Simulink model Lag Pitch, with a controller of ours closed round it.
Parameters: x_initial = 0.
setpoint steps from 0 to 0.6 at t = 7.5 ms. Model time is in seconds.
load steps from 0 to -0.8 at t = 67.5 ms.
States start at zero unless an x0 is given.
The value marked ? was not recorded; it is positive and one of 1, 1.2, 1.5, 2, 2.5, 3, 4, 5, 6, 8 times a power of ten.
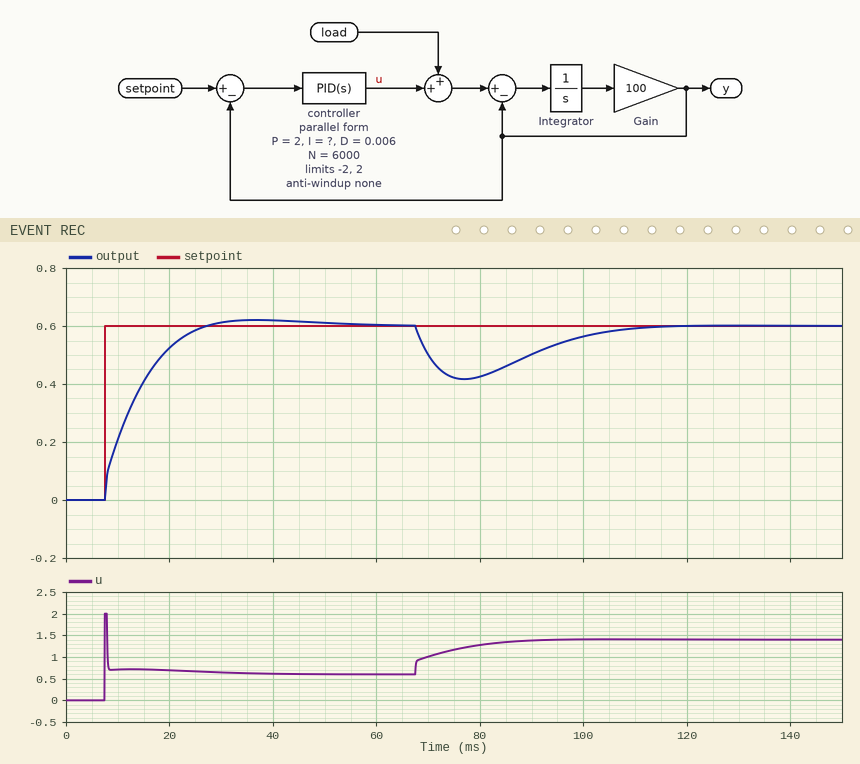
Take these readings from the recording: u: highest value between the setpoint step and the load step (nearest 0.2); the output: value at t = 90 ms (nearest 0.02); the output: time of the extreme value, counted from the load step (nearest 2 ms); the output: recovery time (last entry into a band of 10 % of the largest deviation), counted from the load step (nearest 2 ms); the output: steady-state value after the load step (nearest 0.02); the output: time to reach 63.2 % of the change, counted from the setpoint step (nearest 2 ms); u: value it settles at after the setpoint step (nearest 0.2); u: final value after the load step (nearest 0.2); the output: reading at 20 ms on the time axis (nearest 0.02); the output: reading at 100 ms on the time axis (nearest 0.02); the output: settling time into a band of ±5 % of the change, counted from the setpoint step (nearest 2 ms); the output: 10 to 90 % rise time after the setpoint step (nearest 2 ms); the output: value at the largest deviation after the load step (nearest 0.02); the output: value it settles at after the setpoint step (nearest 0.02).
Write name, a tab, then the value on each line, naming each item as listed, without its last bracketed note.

u: highest value between the setpoint step and the load step	2.0
the output: value at t = 90 ms	0.50
the output: time of the extreme value, counted from the load step	10 ms
the output: recovery time (last entry into a band of 10 % of the largest deviation), counted from the load step	38 ms
the output: steady-state value after the load step	0.60
the output: time to reach 63.2 % of the change, counted from the setpoint step	6 ms
u: value it settles at after the setpoint step	0.6
u: final value after the load step	1.4
the output: reading at 20 ms on the time axis	0.52
the output: reading at 100 ms on the time axis	0.56
the output: settling time into a band of ±5 % of the change, counted from the setpoint step	16 ms
the output: 10 to 90 % rise time after the setpoint step	14 ms
the output: value at the largest deviation after the load step	0.42
the output: value it settles at after the setpoint step	0.60
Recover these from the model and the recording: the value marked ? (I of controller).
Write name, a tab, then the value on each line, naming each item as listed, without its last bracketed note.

the value marked ?	200
